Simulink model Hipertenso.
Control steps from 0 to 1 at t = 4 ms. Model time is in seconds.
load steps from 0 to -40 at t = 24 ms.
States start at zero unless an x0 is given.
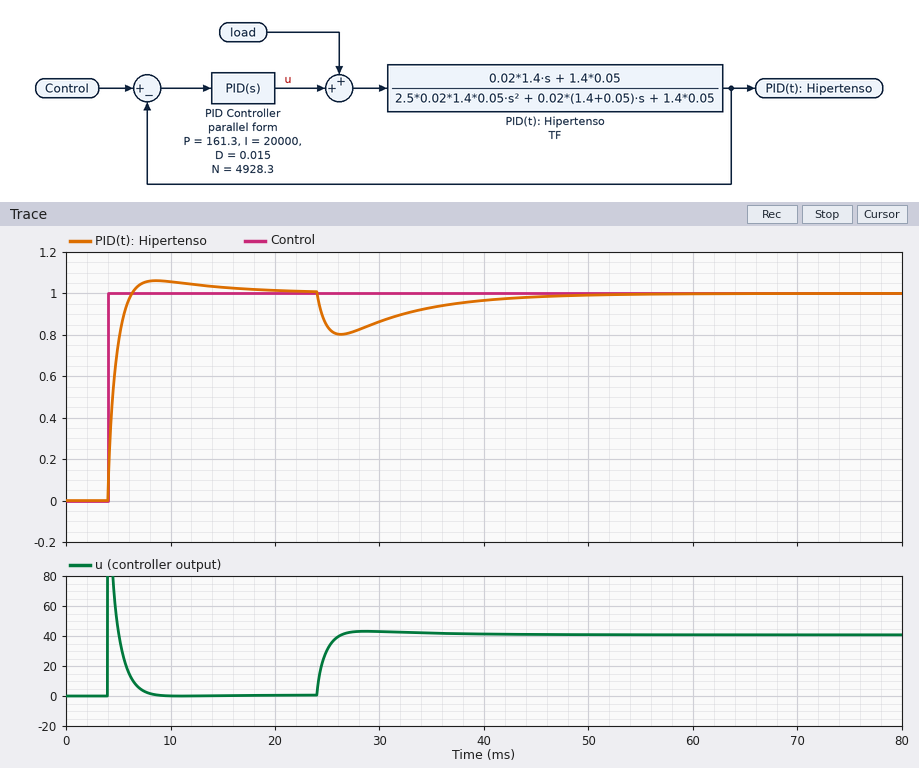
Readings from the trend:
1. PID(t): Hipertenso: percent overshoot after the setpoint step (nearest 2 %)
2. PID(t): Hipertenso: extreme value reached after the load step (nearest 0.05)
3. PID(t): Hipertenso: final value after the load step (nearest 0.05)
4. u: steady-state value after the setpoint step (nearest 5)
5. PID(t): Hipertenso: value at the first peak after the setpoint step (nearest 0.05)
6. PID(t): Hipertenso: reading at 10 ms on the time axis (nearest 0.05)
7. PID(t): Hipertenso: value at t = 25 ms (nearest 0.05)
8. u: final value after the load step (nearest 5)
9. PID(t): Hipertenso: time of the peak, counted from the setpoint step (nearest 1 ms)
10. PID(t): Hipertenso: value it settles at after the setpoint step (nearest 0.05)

6 %
0.80
1.00
0
1.05
1.05
0.85
40
5 ms
1.00
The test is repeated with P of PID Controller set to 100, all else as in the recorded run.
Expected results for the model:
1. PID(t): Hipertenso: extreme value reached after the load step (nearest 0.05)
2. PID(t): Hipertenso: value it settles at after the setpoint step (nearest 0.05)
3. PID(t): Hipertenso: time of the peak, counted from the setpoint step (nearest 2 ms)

0.70
1.00
6 ms
